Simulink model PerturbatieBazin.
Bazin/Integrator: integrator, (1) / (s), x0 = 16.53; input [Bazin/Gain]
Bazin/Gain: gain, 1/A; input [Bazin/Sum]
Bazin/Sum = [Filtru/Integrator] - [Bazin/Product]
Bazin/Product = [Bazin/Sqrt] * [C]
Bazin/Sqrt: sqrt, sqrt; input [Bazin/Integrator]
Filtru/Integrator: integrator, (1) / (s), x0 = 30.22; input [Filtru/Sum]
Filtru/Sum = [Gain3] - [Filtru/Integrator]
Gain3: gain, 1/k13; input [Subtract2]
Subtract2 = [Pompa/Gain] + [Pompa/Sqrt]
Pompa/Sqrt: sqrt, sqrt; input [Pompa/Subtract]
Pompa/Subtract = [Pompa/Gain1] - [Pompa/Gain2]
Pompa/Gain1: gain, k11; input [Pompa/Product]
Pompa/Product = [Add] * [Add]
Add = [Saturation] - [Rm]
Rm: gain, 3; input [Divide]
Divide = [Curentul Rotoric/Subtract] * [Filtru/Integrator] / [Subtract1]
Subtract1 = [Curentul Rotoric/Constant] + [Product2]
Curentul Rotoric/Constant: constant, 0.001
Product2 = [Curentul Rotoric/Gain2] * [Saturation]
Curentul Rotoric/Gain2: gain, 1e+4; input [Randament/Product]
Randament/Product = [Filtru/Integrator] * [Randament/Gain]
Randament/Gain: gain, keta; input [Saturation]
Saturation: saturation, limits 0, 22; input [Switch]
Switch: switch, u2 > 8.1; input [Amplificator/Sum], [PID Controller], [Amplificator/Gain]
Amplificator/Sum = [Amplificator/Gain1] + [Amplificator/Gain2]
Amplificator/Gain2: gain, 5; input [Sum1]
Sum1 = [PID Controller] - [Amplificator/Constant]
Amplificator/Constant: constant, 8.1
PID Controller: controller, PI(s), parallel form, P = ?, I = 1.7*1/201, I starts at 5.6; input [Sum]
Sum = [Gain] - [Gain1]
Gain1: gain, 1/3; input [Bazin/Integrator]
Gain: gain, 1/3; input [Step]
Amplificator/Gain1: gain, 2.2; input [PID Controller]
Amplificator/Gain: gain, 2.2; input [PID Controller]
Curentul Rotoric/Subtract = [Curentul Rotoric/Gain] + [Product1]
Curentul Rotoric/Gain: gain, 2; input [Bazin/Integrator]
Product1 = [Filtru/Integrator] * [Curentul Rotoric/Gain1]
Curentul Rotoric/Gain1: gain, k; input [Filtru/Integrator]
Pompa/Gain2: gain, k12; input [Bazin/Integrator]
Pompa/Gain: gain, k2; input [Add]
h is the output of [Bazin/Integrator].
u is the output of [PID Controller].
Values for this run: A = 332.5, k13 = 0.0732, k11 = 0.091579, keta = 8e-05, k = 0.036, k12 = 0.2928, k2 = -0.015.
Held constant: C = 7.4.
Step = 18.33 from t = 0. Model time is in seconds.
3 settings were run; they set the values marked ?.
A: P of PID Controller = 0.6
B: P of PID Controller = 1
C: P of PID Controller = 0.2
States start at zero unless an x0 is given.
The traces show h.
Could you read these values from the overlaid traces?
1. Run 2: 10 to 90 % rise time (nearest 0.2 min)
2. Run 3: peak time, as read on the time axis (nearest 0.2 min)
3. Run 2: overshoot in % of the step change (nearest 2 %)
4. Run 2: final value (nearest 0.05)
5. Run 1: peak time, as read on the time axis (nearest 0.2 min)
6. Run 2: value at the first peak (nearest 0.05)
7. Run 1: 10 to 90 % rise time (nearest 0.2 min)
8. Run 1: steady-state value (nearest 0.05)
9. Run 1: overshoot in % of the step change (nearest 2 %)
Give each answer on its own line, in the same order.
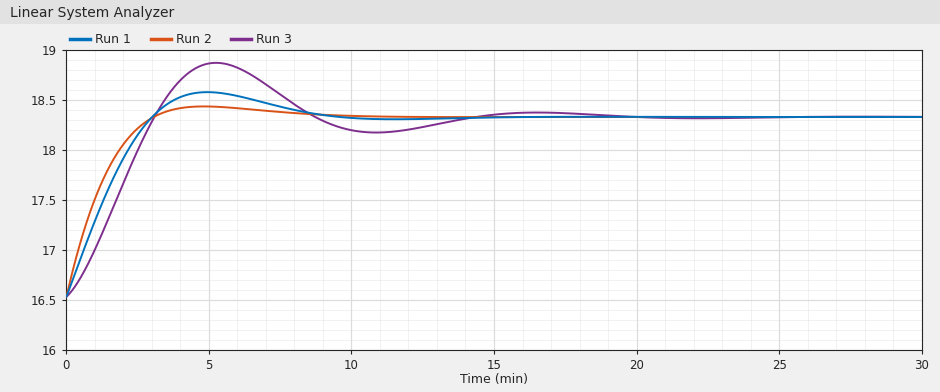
2.2 min
5.2 min
6 %
18.35
5.0 min
18.45
2.2 min
18.35
14 %
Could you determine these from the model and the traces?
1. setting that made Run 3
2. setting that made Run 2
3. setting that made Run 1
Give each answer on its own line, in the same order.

C
B
A
